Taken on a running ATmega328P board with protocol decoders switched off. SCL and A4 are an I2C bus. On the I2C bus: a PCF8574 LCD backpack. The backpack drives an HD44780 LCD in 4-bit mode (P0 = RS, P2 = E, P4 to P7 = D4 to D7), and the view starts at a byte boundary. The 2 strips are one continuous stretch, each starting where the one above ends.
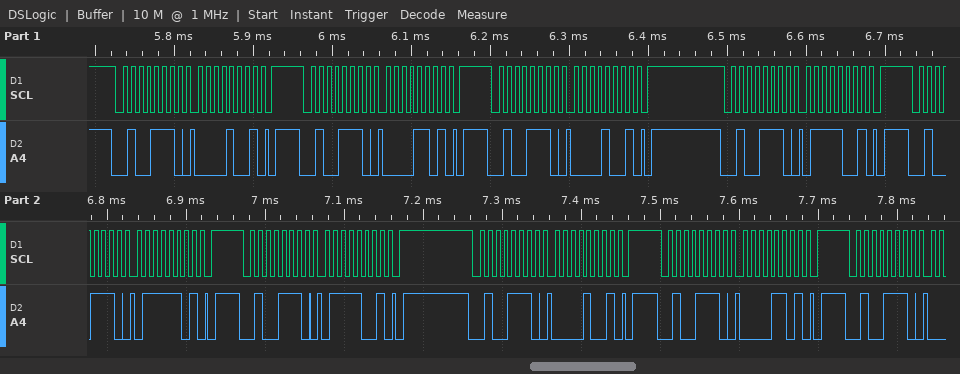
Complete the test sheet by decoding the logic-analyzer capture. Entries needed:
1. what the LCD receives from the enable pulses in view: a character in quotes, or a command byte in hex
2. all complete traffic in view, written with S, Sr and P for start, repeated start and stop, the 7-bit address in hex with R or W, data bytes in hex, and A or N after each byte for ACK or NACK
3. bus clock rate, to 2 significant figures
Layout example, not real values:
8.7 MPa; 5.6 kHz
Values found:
data 0x07; S 27W A 09 A P S 27W A 0D A P S 27W A 09 A P S 27W A 79 A P S 27W A 7D A P S 27W A 79 A P S 27W A 09 A P S 27W A 0D A P S 27W A; 100 kHz
